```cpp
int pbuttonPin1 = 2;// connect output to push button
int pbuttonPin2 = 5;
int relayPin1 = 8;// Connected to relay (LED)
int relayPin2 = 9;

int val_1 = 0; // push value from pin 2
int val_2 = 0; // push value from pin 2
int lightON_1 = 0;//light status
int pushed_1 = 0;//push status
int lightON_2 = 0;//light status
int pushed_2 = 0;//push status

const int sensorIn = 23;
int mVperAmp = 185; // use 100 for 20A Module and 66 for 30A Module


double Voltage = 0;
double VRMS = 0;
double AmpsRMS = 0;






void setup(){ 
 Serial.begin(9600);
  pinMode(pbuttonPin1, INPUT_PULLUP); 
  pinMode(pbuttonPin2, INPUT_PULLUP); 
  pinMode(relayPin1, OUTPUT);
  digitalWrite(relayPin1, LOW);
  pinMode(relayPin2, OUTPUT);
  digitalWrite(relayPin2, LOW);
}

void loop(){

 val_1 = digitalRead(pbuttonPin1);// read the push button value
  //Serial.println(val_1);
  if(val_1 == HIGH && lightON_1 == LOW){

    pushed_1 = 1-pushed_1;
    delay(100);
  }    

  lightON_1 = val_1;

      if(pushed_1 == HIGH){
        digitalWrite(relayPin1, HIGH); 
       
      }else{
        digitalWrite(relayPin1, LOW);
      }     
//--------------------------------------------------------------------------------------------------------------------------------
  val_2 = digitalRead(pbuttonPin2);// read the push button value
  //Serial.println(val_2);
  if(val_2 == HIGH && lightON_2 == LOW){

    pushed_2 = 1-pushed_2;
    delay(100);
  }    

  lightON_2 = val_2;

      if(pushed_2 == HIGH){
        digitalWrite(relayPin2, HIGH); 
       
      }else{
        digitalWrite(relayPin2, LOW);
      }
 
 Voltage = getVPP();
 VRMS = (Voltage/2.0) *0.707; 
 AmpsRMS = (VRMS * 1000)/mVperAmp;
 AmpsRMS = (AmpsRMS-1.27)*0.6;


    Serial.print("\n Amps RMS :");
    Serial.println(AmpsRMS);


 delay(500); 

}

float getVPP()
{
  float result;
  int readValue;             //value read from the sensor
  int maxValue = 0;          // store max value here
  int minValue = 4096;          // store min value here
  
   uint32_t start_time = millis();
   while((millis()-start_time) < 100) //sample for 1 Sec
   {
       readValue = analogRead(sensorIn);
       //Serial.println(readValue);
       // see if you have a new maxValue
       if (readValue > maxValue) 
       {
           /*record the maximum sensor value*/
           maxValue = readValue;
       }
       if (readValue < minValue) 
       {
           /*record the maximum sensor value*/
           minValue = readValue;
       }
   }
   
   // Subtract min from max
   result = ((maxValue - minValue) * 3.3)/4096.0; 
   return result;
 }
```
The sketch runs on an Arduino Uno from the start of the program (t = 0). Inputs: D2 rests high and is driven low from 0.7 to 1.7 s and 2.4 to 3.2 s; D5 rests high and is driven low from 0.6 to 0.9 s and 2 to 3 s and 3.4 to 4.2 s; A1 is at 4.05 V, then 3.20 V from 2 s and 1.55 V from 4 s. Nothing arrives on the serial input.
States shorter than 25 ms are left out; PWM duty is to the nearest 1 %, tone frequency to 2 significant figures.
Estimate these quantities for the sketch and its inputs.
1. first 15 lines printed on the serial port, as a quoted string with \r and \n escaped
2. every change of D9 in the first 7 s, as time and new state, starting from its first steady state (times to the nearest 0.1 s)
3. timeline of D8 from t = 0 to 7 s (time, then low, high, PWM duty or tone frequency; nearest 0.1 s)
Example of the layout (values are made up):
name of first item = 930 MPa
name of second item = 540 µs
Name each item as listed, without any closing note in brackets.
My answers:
first 15 lines printed on the serial port, as a quoted string with \r and \n escaped = "\n Amps RMS :-0.76\r\n\n Amps RMS :-0.76\r\n\n Amps RMS :-0.76\r\n\n Amps RMS :-0.76\r\n\n Amps RMS :-0.76\r\n\n Amps RMS :-0.76\r\n\n Amps RMS :-0.76\r\n\n"
every change of D9 in the first 7 s, as time and new state, starting from its first steady state = 0 s low; 0.2 s high; 1.5 s low; 4.8 s high
timeline of D8 from t = 0 to 7 s = 0 s low; 0.1 s high; 2.2 s low; 3.5 s high
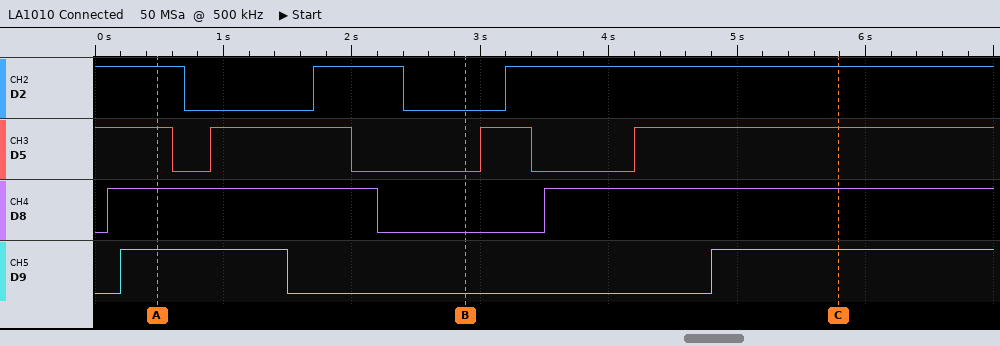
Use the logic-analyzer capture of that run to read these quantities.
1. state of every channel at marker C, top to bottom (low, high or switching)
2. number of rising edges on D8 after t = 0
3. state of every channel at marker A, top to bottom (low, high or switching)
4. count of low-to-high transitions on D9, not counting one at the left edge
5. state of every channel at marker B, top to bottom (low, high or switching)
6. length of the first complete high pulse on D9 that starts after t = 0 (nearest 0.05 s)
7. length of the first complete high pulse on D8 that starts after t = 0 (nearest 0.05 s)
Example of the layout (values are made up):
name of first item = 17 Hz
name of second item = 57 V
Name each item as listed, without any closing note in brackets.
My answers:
state of every channel at marker C, top to bottom = D2 high, D5 high, D8 high, D9 high
number of rising edges on D8 after t = 0 = 2
state of every channel at marker A, top to bottom = D2 high, D5 high, D8 high, D9 high
count of low-to-high transitions on D9, not counting one at the left edge = 2
state of every channel at marker B, top to bottom = D2 low, D5 low, D8 low, D9 low
length of the first complete high pulse on D9 that starts after t = 0 = 1.30 s
length of the first complete high pulse on D8 that starts after t = 0 = 2.10 s
